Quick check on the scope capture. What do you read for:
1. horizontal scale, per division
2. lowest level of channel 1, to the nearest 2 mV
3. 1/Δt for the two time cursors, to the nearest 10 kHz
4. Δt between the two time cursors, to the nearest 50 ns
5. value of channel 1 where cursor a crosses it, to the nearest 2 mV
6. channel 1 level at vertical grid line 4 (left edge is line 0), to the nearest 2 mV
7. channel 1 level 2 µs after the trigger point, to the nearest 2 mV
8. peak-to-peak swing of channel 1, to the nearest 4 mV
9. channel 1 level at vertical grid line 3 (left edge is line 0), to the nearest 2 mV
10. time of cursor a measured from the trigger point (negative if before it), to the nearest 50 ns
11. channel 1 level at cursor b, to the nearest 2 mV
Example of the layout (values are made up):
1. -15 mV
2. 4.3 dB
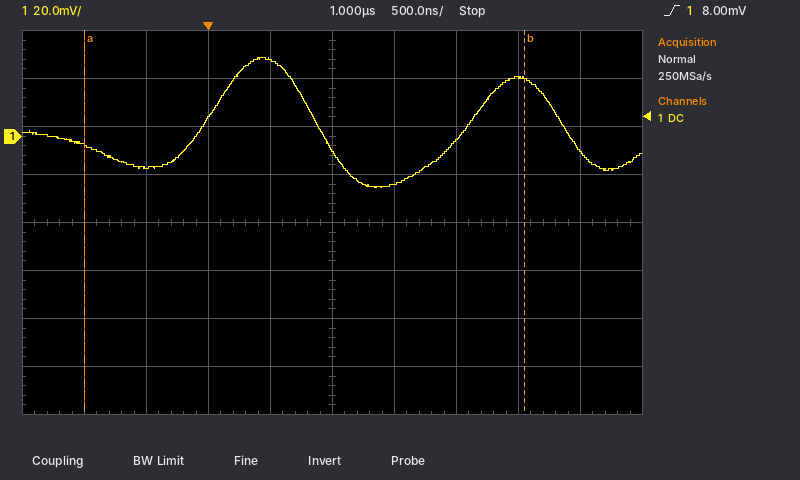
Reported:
1. 500 ns
2. -22 mV
3. 280 kHz
4. 3.55 µs
5. -4 mV
6. 32 mV
7. -2 mV
8. 56 mV
9. 8 mV
10. -1.00 µs
11. 24 mV
